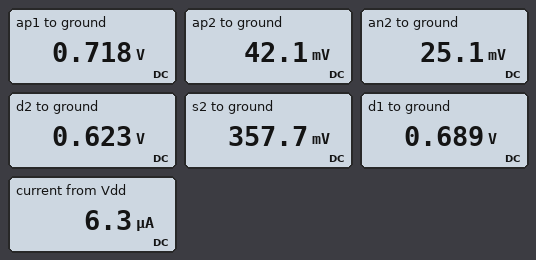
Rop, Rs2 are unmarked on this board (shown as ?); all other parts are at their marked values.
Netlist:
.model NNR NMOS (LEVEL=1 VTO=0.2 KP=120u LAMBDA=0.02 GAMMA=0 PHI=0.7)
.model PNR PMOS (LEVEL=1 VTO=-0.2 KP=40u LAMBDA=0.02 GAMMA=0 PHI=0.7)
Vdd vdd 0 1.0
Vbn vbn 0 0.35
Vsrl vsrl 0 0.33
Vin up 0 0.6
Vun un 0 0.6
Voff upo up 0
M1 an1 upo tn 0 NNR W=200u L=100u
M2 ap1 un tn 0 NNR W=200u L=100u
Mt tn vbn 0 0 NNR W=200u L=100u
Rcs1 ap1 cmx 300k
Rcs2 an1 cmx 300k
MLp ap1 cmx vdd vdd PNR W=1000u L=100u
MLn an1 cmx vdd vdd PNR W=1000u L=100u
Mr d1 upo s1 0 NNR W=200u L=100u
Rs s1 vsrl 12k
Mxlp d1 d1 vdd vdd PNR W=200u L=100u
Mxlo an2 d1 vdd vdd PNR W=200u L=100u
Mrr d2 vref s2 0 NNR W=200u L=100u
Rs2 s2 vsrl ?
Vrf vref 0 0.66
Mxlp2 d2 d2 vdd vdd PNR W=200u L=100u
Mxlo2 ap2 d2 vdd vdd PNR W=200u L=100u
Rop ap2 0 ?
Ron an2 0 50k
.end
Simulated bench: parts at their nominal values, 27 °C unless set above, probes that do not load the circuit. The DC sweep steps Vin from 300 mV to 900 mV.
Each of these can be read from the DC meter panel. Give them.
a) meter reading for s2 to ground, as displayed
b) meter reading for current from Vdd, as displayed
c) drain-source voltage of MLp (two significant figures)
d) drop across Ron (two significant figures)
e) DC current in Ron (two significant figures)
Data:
357.7 mV
6.3 µA
-280 mV
25 mV
500 nA
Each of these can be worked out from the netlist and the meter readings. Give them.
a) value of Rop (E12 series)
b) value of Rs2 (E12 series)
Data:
33 kΩ
22 kΩ
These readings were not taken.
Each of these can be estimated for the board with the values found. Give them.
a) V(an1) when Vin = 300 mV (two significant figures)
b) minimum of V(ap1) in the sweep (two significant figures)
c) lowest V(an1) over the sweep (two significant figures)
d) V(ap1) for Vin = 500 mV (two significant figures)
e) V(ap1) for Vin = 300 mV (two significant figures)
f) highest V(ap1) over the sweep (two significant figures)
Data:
970 mV
440 mV
440 mV
460 mV
440 mV
970 mV
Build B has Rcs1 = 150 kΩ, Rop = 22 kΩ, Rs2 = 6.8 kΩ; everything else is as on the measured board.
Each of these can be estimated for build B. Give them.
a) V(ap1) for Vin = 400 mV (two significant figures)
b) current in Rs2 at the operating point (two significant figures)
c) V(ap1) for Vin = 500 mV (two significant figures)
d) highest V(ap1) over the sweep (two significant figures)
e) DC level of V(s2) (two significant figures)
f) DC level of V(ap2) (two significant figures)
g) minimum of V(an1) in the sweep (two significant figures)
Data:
570 mV
1.7 µA
580 mV
880 mV
340 mV
38 mV
390 mV
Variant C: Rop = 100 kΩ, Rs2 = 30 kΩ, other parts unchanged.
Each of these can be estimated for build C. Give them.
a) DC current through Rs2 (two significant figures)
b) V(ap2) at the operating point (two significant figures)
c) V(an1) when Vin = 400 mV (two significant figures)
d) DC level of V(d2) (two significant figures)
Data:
1.1 µA
110 mV
970 mV
630 mV
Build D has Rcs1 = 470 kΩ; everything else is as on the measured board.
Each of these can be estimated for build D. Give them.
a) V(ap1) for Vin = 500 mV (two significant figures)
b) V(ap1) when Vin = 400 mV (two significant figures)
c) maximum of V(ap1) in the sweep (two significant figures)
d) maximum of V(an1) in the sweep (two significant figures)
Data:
330 mV
290 mV
980 mV
970 mV
